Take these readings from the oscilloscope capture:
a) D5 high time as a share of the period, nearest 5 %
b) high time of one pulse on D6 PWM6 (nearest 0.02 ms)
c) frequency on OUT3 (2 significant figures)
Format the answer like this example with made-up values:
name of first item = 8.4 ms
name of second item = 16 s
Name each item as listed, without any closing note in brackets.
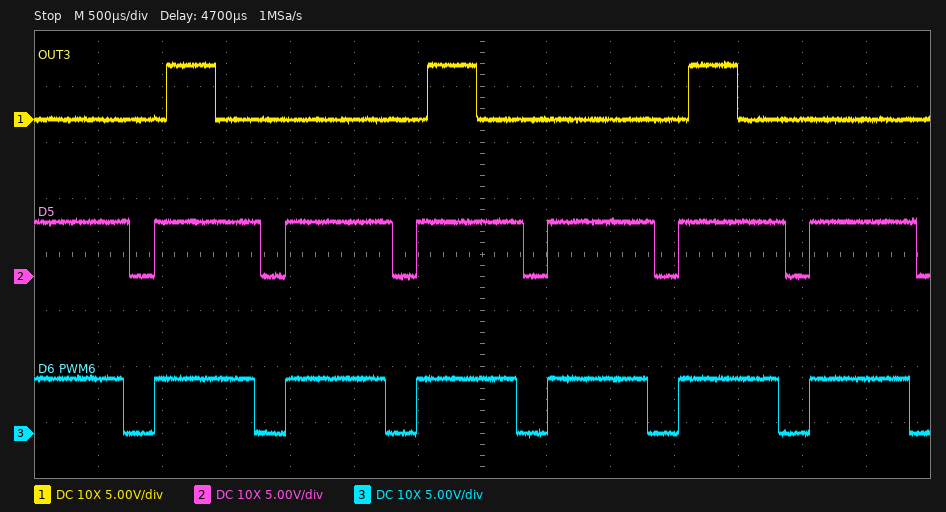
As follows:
D5 high time as a share of the period, nearest 5 % = 80 %
high time of one pulse on D6 PWM6 = 0.78 ms
frequency on OUT3 = 490 Hz
